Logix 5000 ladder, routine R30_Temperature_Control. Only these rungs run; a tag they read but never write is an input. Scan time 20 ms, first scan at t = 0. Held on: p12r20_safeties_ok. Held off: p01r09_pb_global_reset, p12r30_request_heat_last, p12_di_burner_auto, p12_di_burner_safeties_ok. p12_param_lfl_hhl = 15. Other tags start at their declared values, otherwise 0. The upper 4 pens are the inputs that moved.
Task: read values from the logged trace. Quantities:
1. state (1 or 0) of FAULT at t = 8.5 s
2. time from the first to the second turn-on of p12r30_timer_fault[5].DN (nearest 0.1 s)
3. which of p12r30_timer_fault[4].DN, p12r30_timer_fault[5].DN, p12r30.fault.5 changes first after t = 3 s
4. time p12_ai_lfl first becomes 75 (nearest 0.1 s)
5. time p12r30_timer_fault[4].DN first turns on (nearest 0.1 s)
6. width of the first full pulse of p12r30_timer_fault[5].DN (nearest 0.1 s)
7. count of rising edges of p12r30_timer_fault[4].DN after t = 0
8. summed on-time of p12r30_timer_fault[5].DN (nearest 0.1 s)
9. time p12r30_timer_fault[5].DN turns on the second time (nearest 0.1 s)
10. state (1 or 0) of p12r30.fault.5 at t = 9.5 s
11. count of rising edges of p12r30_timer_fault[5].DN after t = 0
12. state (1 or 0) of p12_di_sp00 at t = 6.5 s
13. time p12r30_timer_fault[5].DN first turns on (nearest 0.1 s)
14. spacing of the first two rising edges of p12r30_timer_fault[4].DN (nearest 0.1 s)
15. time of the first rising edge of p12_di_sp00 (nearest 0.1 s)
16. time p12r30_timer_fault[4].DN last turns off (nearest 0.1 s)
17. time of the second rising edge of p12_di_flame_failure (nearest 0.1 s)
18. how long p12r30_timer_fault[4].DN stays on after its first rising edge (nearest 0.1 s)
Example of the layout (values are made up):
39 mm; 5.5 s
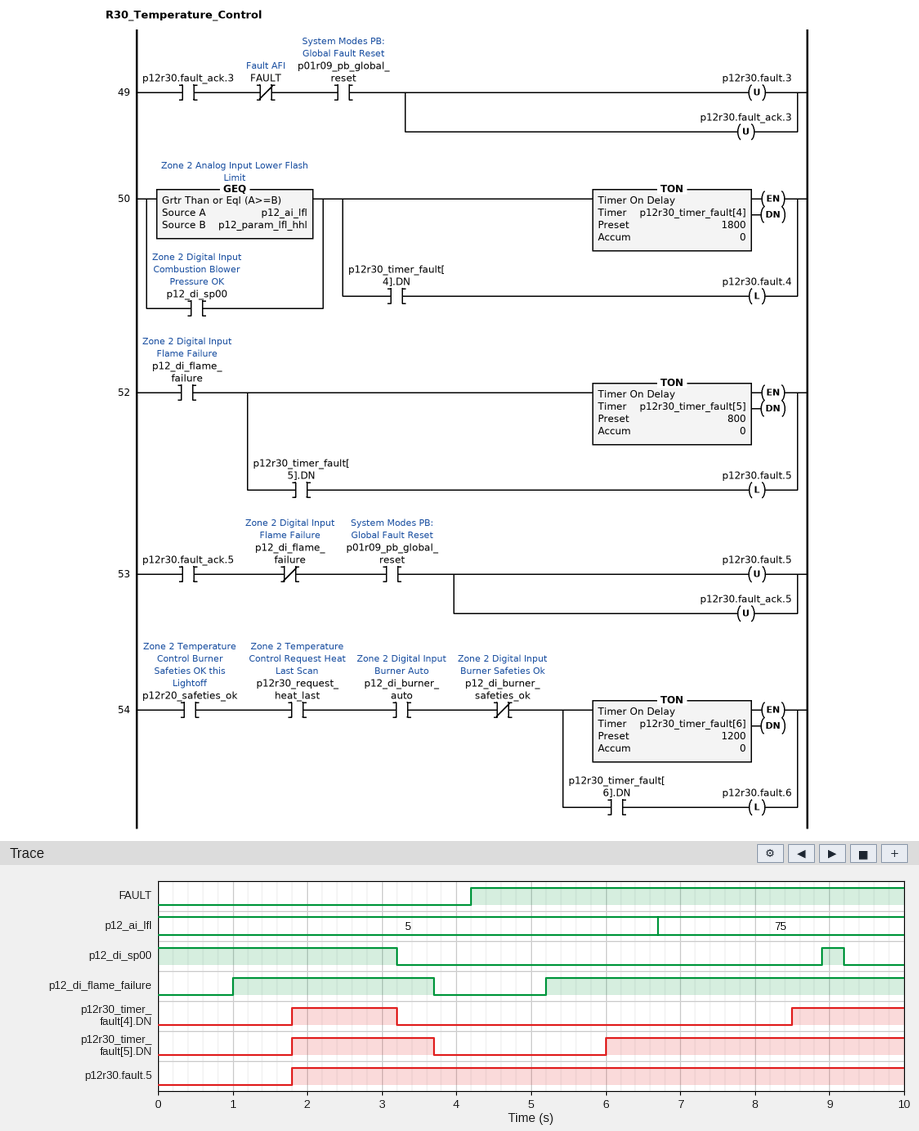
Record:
1; 4.2 s; p12r30_timer_fault[4].DN; 6.7 s; 1.8 s; 1.9 s; 2; 5.9 s; 6.0 s; 1; 2; 0; 1.8 s; 6.7 s; 8.9 s; 3.2 s; 5.2 s; 1.4 s
